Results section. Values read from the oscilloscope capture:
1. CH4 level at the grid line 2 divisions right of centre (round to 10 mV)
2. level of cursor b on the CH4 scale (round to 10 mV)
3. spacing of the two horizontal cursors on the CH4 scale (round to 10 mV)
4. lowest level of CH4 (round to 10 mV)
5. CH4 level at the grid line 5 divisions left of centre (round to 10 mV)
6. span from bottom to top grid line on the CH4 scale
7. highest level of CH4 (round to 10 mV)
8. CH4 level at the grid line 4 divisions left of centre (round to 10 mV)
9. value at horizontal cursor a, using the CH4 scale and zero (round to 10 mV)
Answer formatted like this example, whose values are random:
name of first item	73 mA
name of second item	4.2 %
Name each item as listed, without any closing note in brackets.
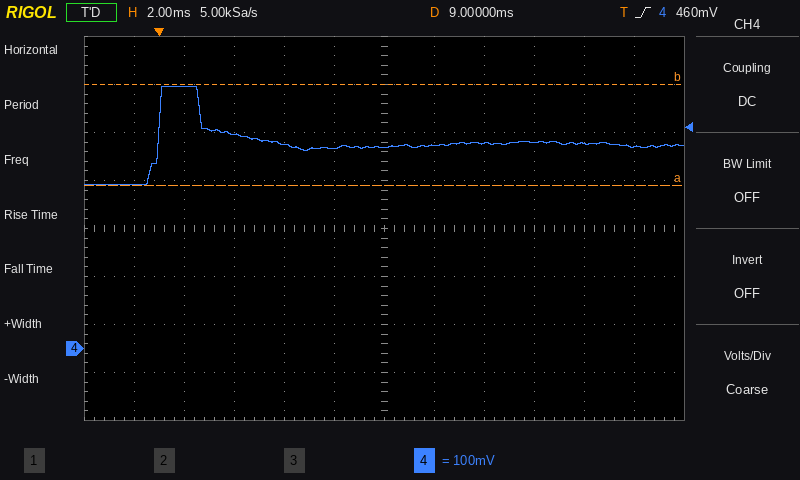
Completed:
CH4 level at the grid line 2 divisions right of centre	430 mV
level of cursor b on the CH4 scale	550 mV
spacing of the two horizontal cursors on the CH4 scale	210 mV
lowest level of CH4	340 mV
CH4 level at the grid line 5 divisions left of centre	340 mV
span from bottom to top grid line on the CH4 scale	800 mV
highest level of CH4	550 mV
CH4 level at the grid line 4 divisions left of centre	550 mV
value at horizontal cursor a, using the CH4 scale and zero	340 mV
